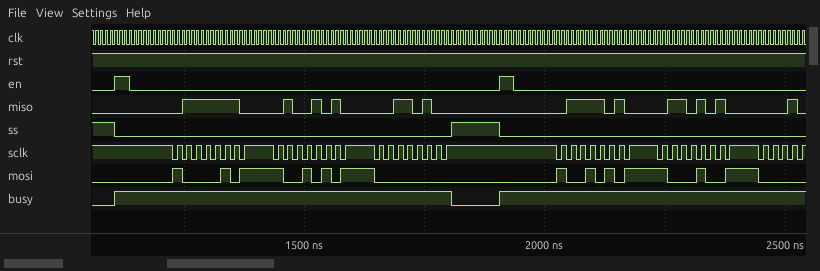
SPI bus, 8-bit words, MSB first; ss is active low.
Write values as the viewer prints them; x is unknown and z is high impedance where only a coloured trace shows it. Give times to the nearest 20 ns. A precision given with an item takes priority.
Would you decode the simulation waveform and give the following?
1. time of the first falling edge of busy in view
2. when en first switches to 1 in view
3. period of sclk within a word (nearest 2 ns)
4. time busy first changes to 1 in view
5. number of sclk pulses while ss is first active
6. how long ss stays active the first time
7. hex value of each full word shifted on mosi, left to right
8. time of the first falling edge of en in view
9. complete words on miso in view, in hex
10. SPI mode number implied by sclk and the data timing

1800 ns
1100 ns
20 ns
1100 ns
24
700 ns
85, 95, 00, 95, 89
1140 ns
7E, 4A, 34, 7A, 6A
3
